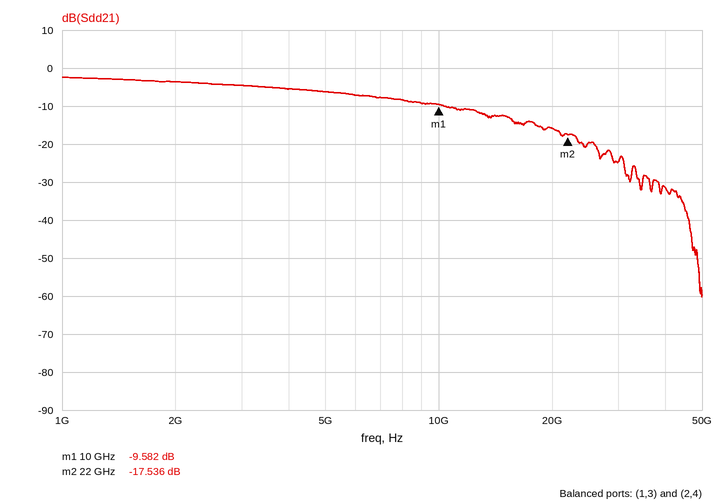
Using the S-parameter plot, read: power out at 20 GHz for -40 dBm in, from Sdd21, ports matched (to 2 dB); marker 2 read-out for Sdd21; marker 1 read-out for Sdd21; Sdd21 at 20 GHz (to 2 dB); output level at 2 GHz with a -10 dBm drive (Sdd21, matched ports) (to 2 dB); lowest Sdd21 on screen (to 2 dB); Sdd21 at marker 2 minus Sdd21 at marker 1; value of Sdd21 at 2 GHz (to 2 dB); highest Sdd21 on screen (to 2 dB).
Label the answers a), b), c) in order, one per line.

a) -56 dBm
b) -17.536 dB
c) -9.582 dB
d) -16 dB
e) -14 dBm
f) -60 dB
g) -7.954 dB
h) -4 dB
i) -2 dB
